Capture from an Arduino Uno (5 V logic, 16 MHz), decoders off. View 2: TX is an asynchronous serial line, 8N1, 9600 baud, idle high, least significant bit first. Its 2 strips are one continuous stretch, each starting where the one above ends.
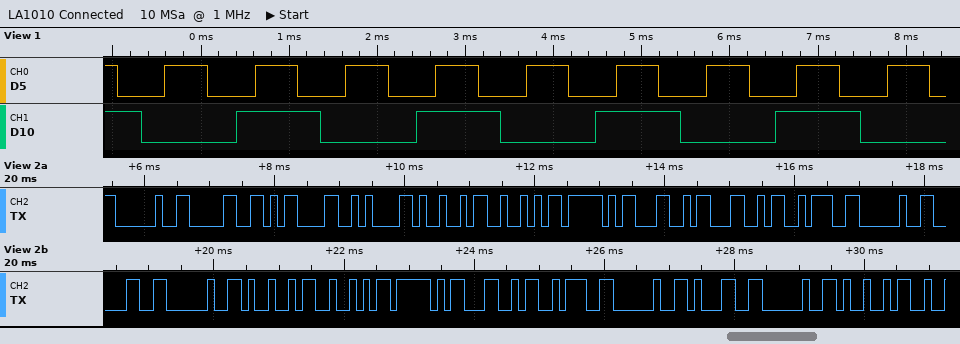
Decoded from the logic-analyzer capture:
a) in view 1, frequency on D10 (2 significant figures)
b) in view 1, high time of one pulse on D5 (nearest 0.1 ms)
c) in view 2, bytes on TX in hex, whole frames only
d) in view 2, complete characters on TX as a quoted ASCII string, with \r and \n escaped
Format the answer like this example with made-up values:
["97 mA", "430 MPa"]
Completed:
["490 Hz", "0.5 ms", "20 30 0D 0A 49 52 5F 4C 4C 3A 20 30 20 49 52 5F 4C 3A 20 31 20 49", "\" 0\\r\\nIR_LL: 0 IR_L: 1 I\""]
